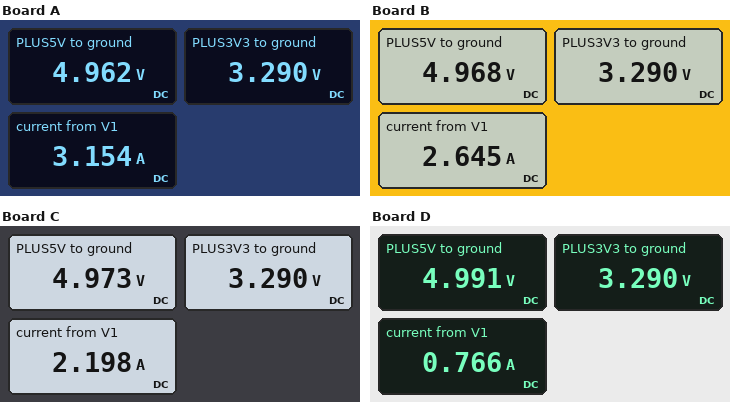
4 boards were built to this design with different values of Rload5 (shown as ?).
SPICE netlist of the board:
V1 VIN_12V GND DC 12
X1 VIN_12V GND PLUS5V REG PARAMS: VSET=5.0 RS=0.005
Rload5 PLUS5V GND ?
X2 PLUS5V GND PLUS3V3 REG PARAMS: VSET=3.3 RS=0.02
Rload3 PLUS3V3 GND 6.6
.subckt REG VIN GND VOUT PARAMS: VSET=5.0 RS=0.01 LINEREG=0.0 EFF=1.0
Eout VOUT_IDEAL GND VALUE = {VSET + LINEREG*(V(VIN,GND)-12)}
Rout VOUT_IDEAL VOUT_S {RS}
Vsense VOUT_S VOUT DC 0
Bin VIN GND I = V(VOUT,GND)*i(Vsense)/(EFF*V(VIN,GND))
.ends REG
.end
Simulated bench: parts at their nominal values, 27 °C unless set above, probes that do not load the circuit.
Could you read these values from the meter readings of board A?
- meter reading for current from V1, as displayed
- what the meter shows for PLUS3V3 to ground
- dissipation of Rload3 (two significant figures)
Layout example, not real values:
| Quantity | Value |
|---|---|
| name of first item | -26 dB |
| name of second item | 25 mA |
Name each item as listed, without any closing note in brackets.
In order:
| Quantity | Value |
|---|---|
| meter reading for current from V1, as displayed | 3.154 A |
| what the meter shows for PLUS3V3 to ground | 3.290 V |
| dissipation of Rload3 | 1.6 W |
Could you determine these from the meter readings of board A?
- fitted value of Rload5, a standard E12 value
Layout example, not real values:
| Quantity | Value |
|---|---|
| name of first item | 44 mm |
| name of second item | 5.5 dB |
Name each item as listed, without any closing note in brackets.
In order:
| Quantity | Value |
|---|---|
| fitted value of Rload5, a standard E12 value | 0.68 Ω |
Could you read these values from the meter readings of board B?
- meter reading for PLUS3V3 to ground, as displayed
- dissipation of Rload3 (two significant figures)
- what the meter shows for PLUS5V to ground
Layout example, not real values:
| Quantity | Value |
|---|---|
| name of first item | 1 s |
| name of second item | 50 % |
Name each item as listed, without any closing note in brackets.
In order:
| Quantity | Value |
|---|---|
| meter reading for PLUS3V3 to ground, as displayed | 3.290 V |
| dissipation of Rload3 | 1.6 W |
| what the meter shows for PLUS5V to ground | 4.968 V |
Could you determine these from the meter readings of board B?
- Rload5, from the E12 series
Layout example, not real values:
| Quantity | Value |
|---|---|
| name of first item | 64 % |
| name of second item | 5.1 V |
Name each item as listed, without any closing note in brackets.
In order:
| Quantity | Value |
|---|---|
| Rload5, from the E12 series | 0.82 Ω |
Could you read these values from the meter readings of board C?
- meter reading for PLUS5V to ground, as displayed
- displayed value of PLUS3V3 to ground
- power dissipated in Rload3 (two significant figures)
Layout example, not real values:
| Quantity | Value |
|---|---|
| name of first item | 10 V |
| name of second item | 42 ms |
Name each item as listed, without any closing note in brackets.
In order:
| Quantity | Value |
|---|---|
| meter reading for PLUS5V to ground, as displayed | 4.973 V |
| displayed value of PLUS3V3 to ground | 3.290 V |
| power dissipated in Rload3 | 1.6 W |
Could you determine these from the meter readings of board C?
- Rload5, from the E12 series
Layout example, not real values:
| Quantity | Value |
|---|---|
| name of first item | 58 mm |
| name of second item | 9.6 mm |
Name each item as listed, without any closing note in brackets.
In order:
| Quantity | Value |
|---|---|
| Rload5, from the E12 series | 1 Ω |
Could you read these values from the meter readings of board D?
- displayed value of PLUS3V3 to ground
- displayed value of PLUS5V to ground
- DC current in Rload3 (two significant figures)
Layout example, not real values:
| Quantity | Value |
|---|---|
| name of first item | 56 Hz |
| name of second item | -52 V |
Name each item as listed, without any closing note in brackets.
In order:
| Quantity | Value |
|---|---|
| displayed value of PLUS3V3 to ground | 3.290 V |
| displayed value of PLUS5V to ground | 4.991 V |
| DC current in Rload3 | 500 mA |
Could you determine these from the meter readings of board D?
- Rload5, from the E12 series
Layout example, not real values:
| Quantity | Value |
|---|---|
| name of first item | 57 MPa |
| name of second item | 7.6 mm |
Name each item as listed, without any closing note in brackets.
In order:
| Quantity | Value |
|---|---|
| Rload5, from the E12 series | 3.3 Ω |
